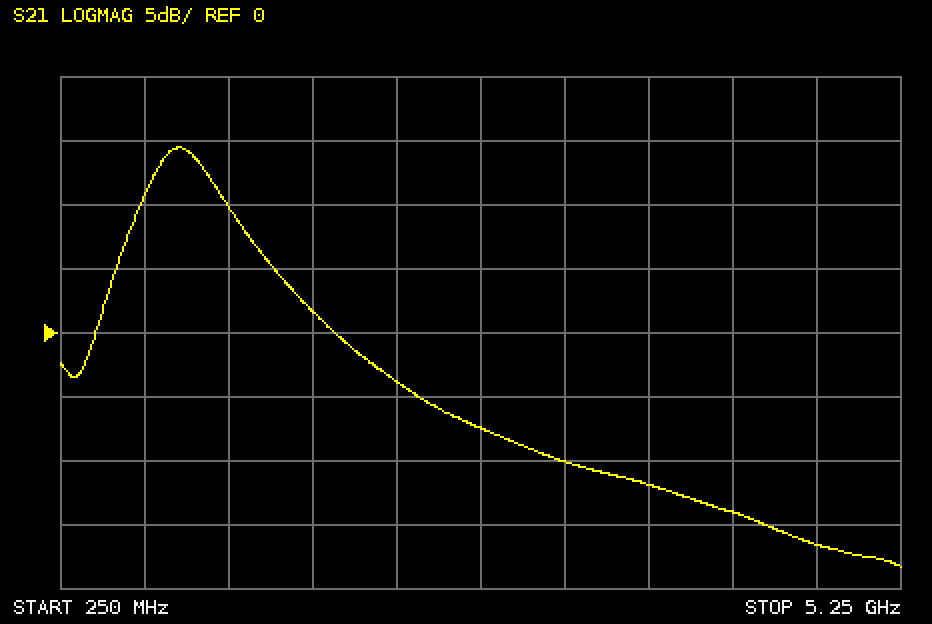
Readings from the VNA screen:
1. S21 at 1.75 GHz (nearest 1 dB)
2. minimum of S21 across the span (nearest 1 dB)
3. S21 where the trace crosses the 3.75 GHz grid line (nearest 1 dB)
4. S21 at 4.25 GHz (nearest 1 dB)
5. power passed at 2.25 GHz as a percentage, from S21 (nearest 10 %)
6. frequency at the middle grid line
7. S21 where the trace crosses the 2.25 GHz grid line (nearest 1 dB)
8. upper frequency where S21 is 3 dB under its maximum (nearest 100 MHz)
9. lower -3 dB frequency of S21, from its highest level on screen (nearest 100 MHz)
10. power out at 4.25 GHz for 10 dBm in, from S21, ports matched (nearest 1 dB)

2 dB
-18 dB
-12 dB
-14 dB
40 %
2.75 GHz
-4 dB
1.2 GHz
800 MHz
-4 dBm
